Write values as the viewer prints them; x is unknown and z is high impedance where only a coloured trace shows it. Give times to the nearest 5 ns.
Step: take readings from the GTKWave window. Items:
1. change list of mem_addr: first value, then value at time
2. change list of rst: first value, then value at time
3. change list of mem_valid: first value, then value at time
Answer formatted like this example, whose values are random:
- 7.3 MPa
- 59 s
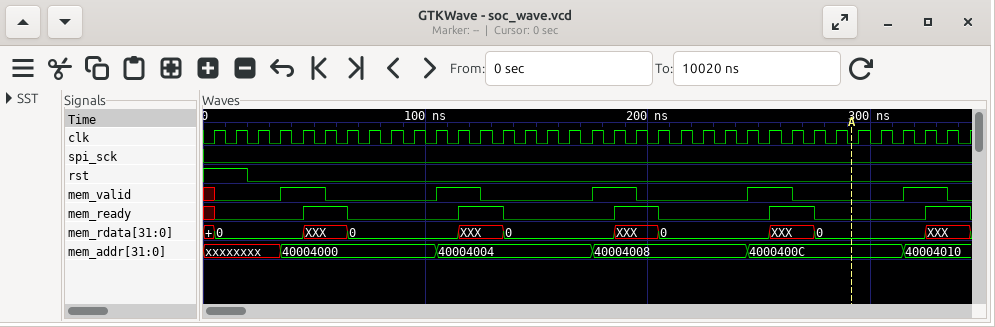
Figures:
- xxxxxxxx, 40004000 at 35 ns, 40004004 at 105 ns, 40004008 at 175 ns, 4000400C at 245 ns, 40004010 at 315 ns
- 1, 0 at 20 ns
- x, 0 at 5 ns, 1 at 35 ns, 0 at 55 ns, 1 at 105 ns, 0 at 125 ns, 1 at 175 ns, 0 at 195 ns, 1 at 245 ns, 0 at 265 ns, 1 at 315 ns, 0 at 335 ns
